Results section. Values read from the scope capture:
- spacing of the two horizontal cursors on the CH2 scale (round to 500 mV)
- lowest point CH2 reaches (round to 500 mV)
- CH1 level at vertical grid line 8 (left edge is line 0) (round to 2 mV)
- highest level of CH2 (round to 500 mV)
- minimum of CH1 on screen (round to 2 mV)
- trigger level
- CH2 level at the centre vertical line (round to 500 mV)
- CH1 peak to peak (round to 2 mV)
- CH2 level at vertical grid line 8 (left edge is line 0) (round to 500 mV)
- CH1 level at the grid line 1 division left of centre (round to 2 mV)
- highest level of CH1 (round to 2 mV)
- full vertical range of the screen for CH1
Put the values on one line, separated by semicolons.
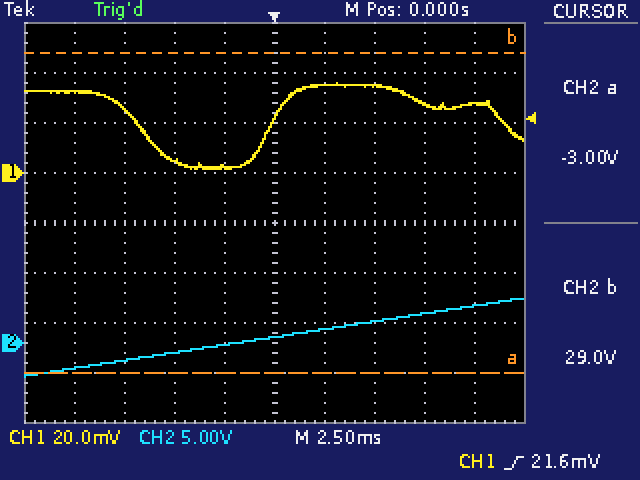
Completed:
32.0 V; -3.5 V; 28 mV; 4.5 V; 2 mV; 21.6 mV; 500 mV; 34 mV; 3.0 V; 2 mV; 36 mV; 160 mV
